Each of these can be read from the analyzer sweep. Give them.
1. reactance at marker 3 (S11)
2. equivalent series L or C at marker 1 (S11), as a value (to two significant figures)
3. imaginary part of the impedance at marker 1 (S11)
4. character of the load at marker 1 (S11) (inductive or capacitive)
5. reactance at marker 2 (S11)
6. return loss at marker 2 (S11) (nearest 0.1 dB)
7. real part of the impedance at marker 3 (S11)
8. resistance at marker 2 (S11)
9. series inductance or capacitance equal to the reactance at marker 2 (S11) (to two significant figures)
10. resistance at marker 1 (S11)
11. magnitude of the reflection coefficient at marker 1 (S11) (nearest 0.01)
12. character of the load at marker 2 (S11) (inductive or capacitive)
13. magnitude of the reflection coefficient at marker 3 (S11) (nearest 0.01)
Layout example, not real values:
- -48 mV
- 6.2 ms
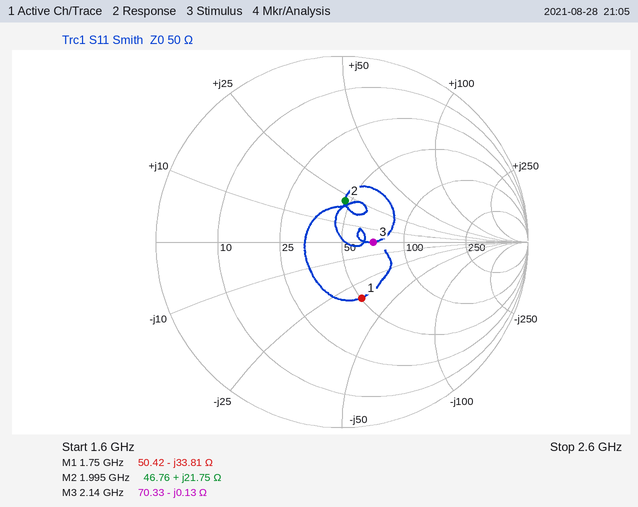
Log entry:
- -0.13 Ω
- 2.7 pF
- -33.81 Ω
- capacitive
- +21.75 Ω
- 13.1 dB
- 70.33 Ω
- 46.76 Ω
- 1.7 nH
- 50.42 Ω
- 0.32
- inductive
- 0.17
